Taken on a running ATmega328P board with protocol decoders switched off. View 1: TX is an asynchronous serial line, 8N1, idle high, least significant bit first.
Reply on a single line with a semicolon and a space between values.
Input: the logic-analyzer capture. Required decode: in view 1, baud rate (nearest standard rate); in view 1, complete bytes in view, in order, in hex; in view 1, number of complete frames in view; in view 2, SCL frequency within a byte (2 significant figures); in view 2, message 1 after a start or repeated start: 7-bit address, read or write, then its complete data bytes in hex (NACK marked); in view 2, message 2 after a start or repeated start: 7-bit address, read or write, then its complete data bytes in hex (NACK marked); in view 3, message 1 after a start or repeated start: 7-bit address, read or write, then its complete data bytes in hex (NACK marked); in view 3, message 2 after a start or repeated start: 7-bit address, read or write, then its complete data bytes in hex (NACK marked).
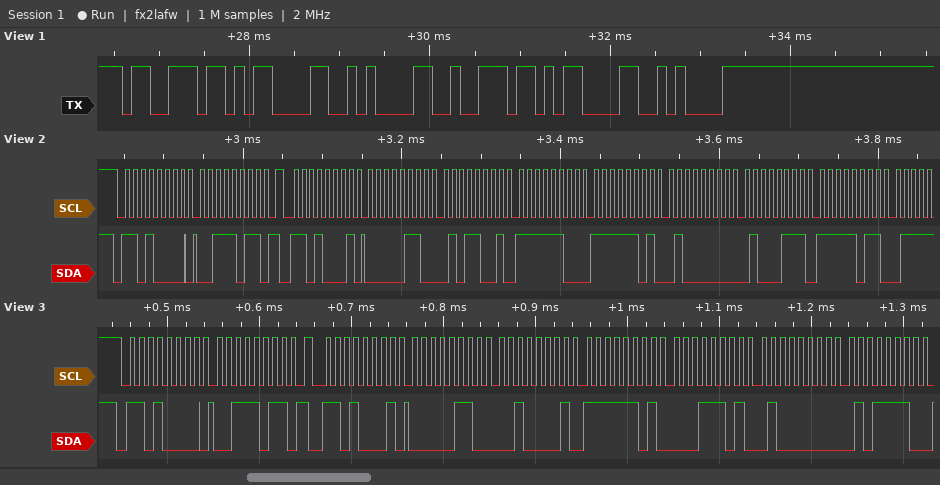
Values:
9600 baud; 73 0D 0A 72 0D 0A; 6; 100 kHz; 0x68 write: 3B; 0x68 read: 06 59 FC FD 40 47 FB; 0x68 write: 3B; 0x68 read: 06 21 FD 1D 40 5E
